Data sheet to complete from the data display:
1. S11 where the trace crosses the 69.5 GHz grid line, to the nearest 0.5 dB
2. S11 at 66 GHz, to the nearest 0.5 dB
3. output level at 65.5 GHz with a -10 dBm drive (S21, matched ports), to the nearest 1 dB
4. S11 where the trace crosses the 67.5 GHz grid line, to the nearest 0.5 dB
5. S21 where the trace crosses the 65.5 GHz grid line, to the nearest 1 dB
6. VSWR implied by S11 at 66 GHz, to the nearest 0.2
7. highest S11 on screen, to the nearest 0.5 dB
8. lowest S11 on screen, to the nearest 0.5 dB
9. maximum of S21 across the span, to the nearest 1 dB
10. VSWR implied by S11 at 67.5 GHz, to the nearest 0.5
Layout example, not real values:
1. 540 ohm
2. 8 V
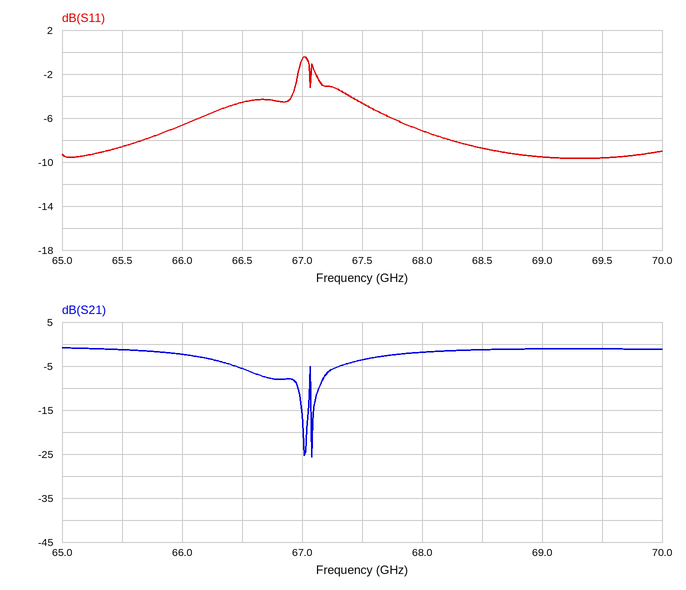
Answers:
1. -9.5 dB
2. -6.5 dB
3. -11 dBm
4. -4.5 dB
5. -1 dB
6. 2.8
7. -0.5 dB
8. -9.5 dB
9. -1 dB
10. 4.0
